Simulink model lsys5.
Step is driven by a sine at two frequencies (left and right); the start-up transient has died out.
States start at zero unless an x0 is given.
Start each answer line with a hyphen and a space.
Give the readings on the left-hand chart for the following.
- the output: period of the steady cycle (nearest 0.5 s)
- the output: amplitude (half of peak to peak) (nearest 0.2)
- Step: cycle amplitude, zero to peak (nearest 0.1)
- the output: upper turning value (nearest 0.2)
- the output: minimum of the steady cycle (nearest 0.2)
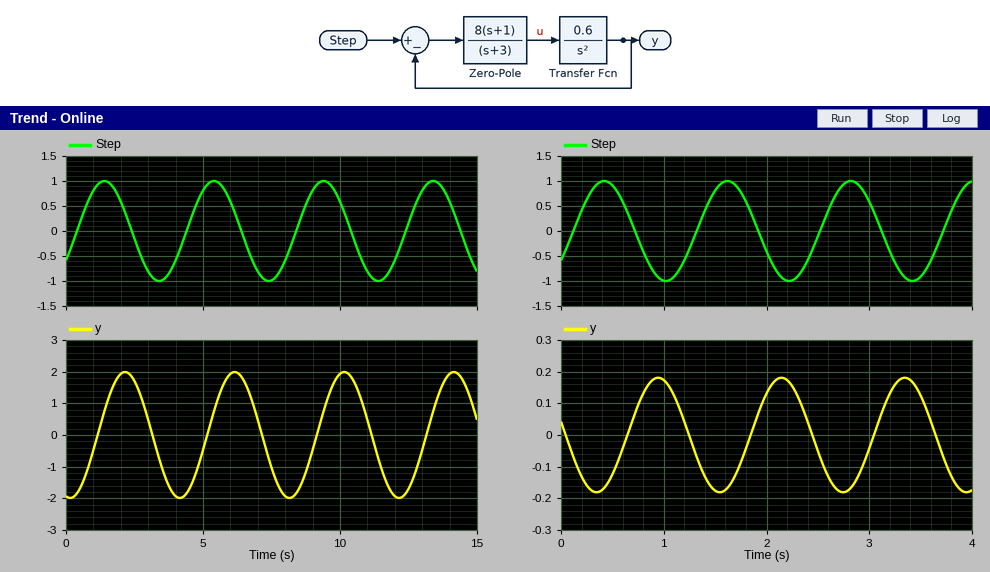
- 4.0 s
- 2.0
- 1.0
- 2.0
- -2.0
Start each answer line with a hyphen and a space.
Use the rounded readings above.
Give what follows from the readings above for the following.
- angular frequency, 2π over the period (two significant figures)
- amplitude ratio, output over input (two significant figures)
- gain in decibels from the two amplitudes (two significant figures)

- 1.6 rad/s
- 2.0
- 6.0 dB
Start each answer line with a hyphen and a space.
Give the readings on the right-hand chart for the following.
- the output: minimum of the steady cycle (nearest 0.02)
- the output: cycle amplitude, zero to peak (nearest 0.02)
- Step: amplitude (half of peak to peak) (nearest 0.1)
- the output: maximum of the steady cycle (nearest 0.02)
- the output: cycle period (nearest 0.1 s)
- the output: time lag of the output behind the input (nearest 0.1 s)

- -0.18
- 0.18
- 1.0
- 0.18
- 1.2 s
- 0.5 s
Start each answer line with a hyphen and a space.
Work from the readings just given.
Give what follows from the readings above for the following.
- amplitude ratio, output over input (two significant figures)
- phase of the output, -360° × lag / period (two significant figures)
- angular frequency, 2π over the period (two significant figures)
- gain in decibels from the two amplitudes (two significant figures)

- 0.18
- -150°
- 5.2 rad/s
- -15 dB
